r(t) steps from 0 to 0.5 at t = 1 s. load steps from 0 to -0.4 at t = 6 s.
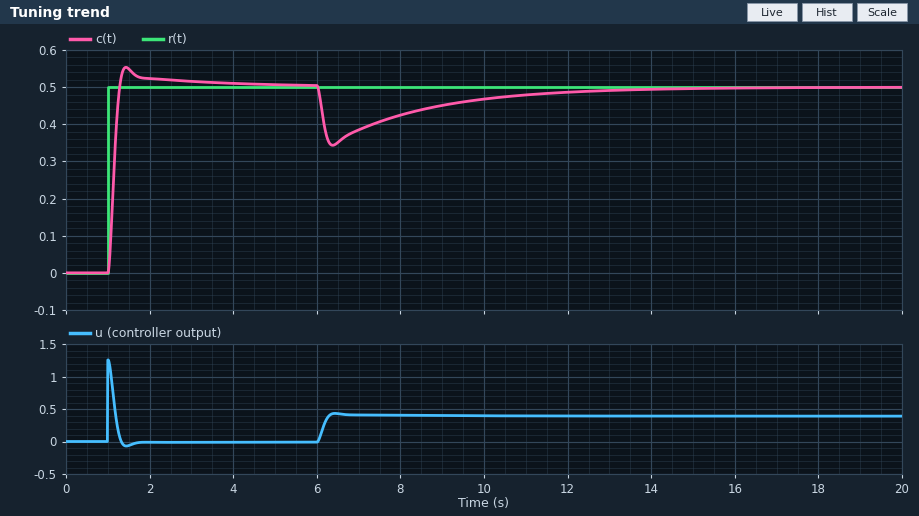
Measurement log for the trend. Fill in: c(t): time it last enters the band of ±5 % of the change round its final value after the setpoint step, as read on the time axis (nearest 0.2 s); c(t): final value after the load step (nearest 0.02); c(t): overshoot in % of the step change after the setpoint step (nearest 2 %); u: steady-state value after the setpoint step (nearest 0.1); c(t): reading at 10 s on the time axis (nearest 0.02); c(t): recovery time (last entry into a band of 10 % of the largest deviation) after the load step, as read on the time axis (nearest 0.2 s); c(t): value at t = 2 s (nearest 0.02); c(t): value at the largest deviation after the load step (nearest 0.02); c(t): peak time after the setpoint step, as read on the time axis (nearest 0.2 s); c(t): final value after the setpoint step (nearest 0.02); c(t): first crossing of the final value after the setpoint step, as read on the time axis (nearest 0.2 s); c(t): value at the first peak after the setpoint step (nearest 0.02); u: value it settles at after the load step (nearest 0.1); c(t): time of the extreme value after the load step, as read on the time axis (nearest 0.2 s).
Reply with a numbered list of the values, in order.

1. 1.8 s
2. 0.50
3. 10 %
4. 0.0
5. 0.46
6. 11.6 s
7. 0.52
8. 0.34
9. 1.4 s
10. 0.50
11. 1.2 s
12. 0.56
13. 0.4
14. 6.4 s
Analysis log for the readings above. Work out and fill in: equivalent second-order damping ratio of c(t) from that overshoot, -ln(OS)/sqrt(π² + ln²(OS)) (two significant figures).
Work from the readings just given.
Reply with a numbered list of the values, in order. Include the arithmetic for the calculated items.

1. ln(0.1) = -2.303; 2.303 / sqrt(9.870 + 5.302) = 0.59
